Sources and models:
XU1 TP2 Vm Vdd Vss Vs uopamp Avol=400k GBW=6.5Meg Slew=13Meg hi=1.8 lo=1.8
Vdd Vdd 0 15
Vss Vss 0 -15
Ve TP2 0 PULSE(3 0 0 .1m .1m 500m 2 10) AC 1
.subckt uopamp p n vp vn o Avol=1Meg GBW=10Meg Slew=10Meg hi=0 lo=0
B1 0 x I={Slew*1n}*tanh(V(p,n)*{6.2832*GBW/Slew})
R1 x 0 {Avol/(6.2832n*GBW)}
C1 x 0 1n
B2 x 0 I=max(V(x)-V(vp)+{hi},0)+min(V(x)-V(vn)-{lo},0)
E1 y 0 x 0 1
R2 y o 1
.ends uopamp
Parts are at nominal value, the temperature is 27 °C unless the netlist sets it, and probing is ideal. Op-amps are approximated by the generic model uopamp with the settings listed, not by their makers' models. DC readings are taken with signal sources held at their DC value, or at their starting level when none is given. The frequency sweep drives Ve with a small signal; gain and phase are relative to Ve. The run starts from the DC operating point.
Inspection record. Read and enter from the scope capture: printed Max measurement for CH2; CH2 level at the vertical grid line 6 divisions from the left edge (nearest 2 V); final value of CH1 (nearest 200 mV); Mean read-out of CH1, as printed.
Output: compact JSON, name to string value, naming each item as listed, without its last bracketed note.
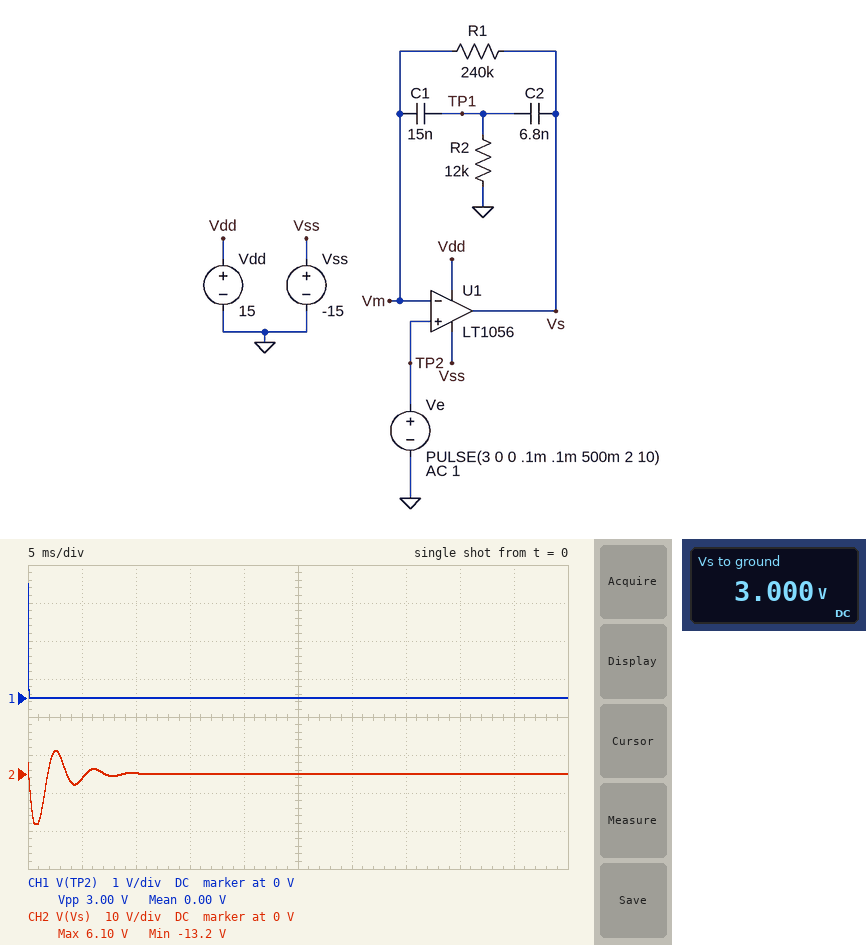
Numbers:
{"printed Max measurement for CH2": "6.10 V", "CH2 level at the vertical grid line 6 divisions from the left edge": "0 V", "final value of CH1": "0 V", "Mean read-out of CH1, as printed": "0.00 V"}
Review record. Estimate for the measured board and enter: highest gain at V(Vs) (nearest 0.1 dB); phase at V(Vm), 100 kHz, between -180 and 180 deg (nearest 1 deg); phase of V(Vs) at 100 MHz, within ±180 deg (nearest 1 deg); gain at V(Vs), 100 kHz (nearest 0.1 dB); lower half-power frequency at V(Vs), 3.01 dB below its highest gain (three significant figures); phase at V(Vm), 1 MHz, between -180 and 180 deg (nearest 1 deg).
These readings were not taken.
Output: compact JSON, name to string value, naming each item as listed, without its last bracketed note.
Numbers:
{"highest gain at V(Vs)": "23.4 dB", "phase at V(Vm), 100 kHz, between -180 and 180 deg": "-1 deg", "phase of V(Vs) at 100 MHz, within ±180 deg": "-86 deg", "gain at V(Vs), 100 kHz": "0 dB", "lower half-power frequency at V(Vs), 3.01 dB below its highest gain": "231 Hz", "phase at V(Vm), 1 MHz, between -180 and 180 deg": "-9 deg"}
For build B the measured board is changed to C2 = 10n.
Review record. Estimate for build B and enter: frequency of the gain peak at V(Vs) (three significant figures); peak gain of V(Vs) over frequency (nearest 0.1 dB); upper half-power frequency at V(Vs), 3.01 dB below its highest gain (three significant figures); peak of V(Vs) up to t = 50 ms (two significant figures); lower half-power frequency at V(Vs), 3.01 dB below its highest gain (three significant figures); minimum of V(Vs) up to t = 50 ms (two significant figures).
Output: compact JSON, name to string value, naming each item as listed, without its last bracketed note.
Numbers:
{"frequency of the gain peak at V(Vs)": "242 Hz", "peak gain of V(Vs) over frequency": "22.3 dB", "upper half-power frequency at V(Vs), 3.01 dB below its highest gain": "304 Hz", "peak of V(Vs) up to t = 50 ms": "5.7 V", "lower half-power frequency at V(Vs), 3.01 dB below its highest gain": "193 Hz", "minimum of V(Vs) up to t = 50 ms": "-12 V"}
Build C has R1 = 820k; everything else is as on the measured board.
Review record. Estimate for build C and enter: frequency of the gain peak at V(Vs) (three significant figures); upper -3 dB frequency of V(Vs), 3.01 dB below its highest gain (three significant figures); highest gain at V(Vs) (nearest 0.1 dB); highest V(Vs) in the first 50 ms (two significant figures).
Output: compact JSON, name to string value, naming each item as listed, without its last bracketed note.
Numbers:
{"frequency of the gain peak at V(Vs)": "159 Hz", "upper -3 dB frequency of V(Vs), 3.01 dB below its highest gain": "181 Hz", "highest gain at V(Vs)": "33.6 dB", "highest V(Vs) in the first 50 ms": "8.8 V"}
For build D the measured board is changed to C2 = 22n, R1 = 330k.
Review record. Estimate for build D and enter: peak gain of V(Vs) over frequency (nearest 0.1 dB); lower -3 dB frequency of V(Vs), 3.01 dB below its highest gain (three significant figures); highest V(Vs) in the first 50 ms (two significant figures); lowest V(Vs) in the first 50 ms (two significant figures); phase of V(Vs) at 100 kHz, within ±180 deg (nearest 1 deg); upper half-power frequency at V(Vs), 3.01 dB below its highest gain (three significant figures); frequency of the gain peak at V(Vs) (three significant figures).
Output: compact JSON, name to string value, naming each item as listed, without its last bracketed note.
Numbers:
{"peak gain of V(Vs) over frequency": "21.7 dB", "lower -3 dB frequency of V(Vs), 3.01 dB below its highest gain": "115 Hz", "highest V(Vs) in the first 50 ms": "5.3 V", "lowest V(Vs) in the first 50 ms": "-9.9 V", "phase of V(Vs) at 100 kHz, within ±180 deg": "-1 deg", "upper half-power frequency at V(Vs), 3.01 dB below its highest gain": "169 Hz", "frequency of the gain peak at V(Vs)": "139 Hz"}
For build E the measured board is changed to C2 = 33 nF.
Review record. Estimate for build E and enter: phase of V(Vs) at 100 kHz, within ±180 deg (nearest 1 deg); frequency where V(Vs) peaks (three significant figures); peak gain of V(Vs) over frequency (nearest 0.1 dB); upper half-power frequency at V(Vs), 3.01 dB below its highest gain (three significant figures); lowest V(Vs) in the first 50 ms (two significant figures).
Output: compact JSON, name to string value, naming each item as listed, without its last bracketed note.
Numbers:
{"phase of V(Vs) at 100 kHz, within ±180 deg": "-1 deg", "frequency where V(Vs) peaks": "133 Hz", "peak gain of V(Vs) over frequency": "17.2 dB", "upper half-power frequency at V(Vs), 3.01 dB below its highest gain": "170 Hz", "lowest V(Vs) in the first 50 ms": "-6.5 V"}
